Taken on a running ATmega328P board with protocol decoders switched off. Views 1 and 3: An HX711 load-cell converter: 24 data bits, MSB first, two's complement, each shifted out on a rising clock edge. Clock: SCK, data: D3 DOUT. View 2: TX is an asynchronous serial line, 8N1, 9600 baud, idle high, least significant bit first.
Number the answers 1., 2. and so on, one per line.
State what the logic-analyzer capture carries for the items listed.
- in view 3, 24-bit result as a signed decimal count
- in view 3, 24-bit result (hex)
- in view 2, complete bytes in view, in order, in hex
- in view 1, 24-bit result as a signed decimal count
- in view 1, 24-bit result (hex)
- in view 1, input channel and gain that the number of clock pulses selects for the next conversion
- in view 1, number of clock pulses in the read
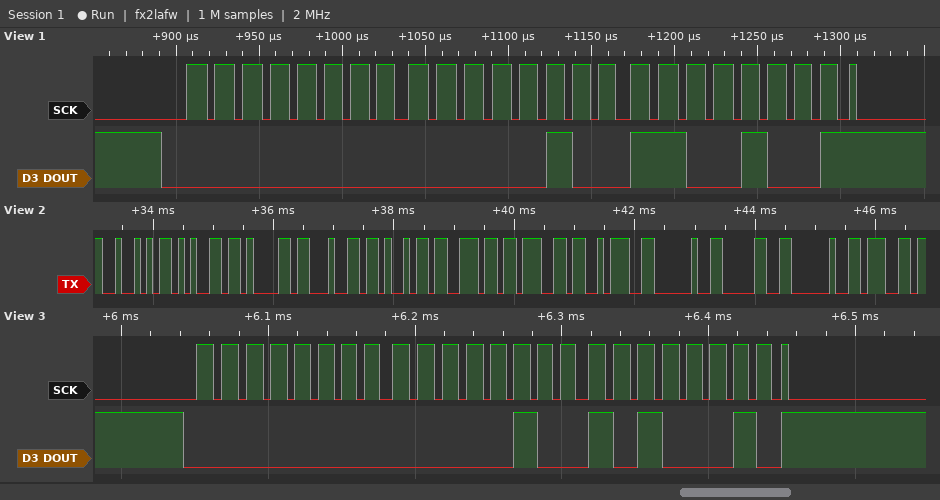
1. 1186
2. 0x0004A2
3. 0x52 0x65 0x61 0x64 0x69 0x6E 0x67 0x3A 0x20 0x30 0x20 0x67
4. 1225
5. 0x0004C9
6. channel A, gain 128
7. 25
